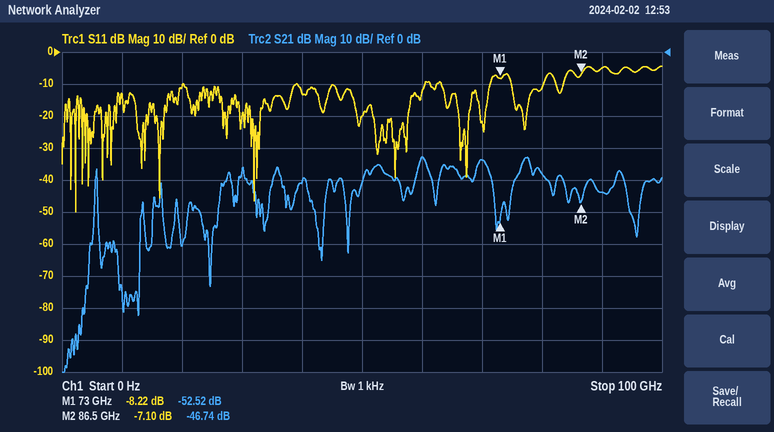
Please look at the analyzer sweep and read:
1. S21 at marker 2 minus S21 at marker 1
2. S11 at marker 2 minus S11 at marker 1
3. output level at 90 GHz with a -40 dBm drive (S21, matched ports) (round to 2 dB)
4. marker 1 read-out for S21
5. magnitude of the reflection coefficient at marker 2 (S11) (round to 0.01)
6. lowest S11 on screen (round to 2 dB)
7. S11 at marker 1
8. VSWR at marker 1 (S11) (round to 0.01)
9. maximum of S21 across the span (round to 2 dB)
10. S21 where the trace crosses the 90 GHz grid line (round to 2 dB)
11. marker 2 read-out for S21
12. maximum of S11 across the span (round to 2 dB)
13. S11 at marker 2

5.78 dB
1.12 dB
-84 dBm
-52.52 dB
0.44
-50 dB
-8.22 dB
2.27
-32 dB
-44 dB
-46.74 dB
-4 dB
-7.10 dB
